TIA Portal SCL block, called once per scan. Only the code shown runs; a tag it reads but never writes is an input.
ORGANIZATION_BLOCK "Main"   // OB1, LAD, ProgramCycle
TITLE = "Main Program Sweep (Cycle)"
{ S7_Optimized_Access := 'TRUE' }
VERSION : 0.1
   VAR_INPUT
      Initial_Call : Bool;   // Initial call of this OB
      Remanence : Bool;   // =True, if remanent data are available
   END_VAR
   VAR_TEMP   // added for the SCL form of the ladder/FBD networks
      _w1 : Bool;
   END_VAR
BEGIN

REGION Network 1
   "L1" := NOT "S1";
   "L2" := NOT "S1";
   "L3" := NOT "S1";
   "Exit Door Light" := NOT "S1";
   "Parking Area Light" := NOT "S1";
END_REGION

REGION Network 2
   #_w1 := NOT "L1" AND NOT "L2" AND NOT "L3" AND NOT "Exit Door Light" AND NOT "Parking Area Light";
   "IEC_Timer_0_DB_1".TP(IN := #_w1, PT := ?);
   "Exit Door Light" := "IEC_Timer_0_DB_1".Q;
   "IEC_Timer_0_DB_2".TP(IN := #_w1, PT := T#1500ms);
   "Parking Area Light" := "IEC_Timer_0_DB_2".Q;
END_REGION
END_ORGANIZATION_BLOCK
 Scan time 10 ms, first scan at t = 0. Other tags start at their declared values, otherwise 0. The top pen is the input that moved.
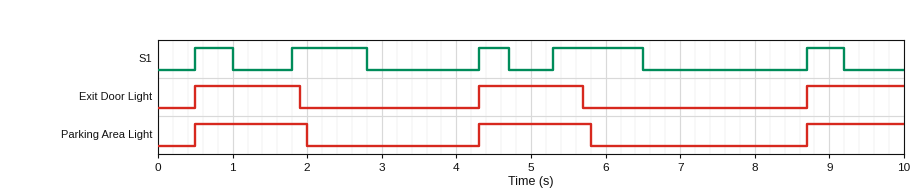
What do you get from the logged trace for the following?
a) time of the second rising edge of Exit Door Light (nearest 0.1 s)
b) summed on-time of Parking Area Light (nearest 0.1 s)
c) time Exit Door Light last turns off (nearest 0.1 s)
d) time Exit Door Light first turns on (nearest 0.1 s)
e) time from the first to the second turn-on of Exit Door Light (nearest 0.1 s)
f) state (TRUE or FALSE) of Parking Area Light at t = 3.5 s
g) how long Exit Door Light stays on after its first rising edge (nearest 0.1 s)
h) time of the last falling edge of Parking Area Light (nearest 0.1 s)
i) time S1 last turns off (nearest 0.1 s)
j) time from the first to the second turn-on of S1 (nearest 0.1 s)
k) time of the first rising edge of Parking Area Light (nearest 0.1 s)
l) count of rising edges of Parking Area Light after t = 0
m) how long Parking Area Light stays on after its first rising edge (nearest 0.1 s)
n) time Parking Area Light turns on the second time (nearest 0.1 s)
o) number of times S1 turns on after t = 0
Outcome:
4.3 s
4.3 s
5.7 s
0.5 s
3.8 s
FALSE
1.4 s
5.8 s
9.2 s
1.3 s
0.5 s
3
1.5 s
4.3 s
5
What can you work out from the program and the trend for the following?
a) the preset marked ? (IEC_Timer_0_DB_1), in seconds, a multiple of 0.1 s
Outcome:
1.4 s
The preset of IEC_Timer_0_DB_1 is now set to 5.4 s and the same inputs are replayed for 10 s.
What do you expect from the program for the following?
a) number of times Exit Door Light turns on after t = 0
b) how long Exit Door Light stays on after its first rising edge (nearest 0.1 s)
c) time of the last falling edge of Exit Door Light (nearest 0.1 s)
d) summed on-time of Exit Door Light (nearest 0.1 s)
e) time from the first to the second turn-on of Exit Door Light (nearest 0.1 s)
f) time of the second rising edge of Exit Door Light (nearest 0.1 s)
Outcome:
2
5.4 s
5.9 s
6.7 s
8.2 s
8.7 s
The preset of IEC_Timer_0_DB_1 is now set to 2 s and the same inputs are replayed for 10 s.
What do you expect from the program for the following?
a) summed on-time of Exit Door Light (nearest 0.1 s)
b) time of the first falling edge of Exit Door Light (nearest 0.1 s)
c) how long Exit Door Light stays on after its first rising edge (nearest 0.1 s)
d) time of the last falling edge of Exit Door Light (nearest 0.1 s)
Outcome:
5.3 s
2.5 s
2.0 s
6.3 s
